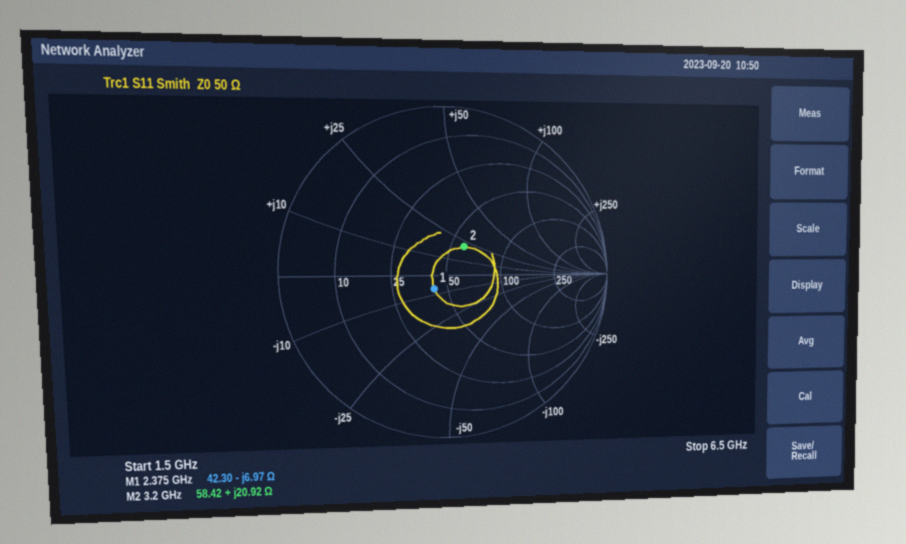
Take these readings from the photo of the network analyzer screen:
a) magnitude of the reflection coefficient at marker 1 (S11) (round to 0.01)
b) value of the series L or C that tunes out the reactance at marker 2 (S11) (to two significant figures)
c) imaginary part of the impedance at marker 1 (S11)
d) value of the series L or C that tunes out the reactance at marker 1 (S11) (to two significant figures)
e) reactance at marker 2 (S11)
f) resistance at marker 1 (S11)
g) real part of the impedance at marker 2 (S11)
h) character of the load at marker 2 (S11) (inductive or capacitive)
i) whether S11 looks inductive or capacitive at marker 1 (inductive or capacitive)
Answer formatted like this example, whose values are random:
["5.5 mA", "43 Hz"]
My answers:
["0.11", "2.4 pF", "-6.97 Ω", "470 pH", "+20.92 Ω", "42.30 Ω", "58.42 Ω", "inductive", "capacitive"]
